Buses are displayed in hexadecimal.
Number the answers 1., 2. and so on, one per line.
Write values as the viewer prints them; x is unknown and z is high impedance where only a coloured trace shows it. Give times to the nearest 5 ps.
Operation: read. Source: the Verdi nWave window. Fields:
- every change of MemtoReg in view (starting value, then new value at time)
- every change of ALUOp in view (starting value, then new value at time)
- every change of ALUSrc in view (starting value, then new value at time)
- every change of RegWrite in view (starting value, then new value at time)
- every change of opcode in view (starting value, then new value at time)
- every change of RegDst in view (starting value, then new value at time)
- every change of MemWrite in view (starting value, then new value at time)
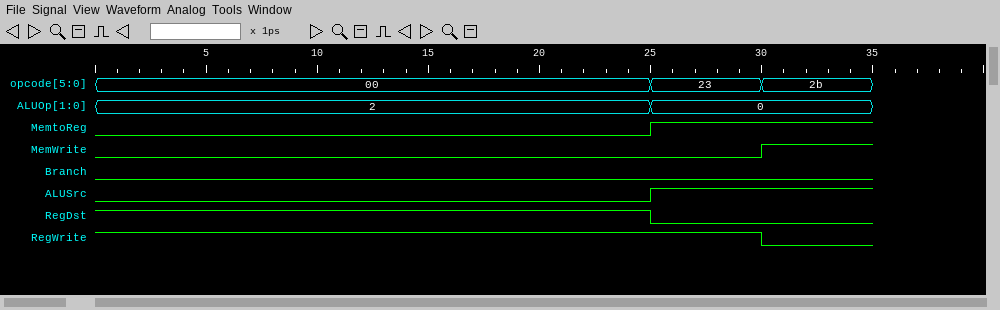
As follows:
1. 0, 1 at 25 ps
2. 2, 0 at 25 ps
3. 0, 1 at 25 ps
4. 1, 0 at 30 ps
5. 00, 23 at 25 ps, 2b at 30 ps
6. 1, 0 at 25 ps
7. 0, 1 at 30 ps
